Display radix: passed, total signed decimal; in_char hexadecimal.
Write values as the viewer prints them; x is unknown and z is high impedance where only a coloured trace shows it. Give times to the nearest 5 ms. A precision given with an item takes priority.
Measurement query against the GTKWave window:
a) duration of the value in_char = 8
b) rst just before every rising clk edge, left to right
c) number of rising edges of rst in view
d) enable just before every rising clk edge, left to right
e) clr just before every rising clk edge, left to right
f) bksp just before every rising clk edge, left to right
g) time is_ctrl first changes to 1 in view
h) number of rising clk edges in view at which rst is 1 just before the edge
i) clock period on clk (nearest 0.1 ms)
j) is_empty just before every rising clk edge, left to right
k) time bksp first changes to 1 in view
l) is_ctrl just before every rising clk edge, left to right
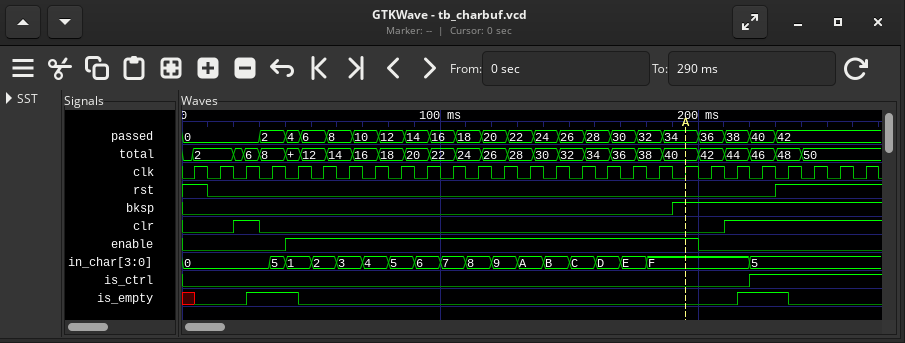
10 ms
1 0 0 0 0 0 0 0 0 0 0 0 0 0 0 0 0 0 0 0 0 0 0 1 1 1 1
1
0 0 0 0 1 1 1 1 1 1 1 1 1 1 1 1 1 1 1 1 0 0 0 0 0 0 0
0 0 1 0 0 0 0 0 0 0 0 0 0 0 0 0 0 0 0 0 0 1 1 1 1 1 1
0 0 0 0 0 0 0 0 0 0 0 0 0 0 0 0 0 0 0 1 1 1 1 1 1 1 1
220 ms
5
10 ms
x 0 0 1 1 0 0 0 0 0 0 0 0 0 0 0 0 0 0 0 0 0 1 1 0 0 0
190 ms
0 0 0 0 0 0 0 0 0 0 0 0 0 0 0 0 0 0 0 0 0 0 1 1 1 1 1
